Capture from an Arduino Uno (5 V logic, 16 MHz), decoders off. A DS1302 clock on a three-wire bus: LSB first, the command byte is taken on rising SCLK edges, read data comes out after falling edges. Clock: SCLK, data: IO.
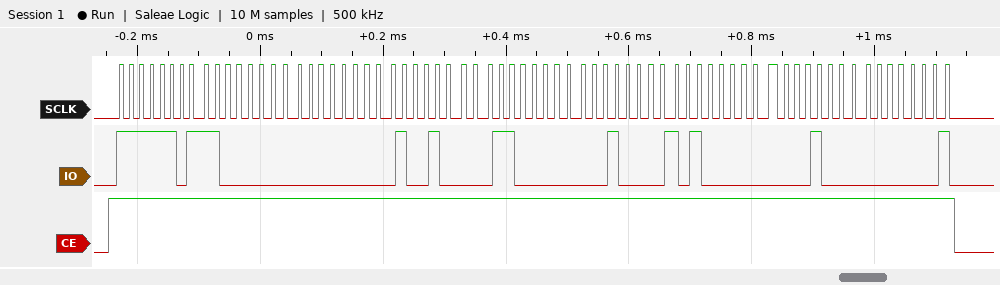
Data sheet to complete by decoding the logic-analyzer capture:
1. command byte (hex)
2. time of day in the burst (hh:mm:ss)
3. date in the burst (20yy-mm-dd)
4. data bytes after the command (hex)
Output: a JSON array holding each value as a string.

["0xBF", "12:00:03", "2010-08-06", "03 00 12 06 08 05 10 80"]
